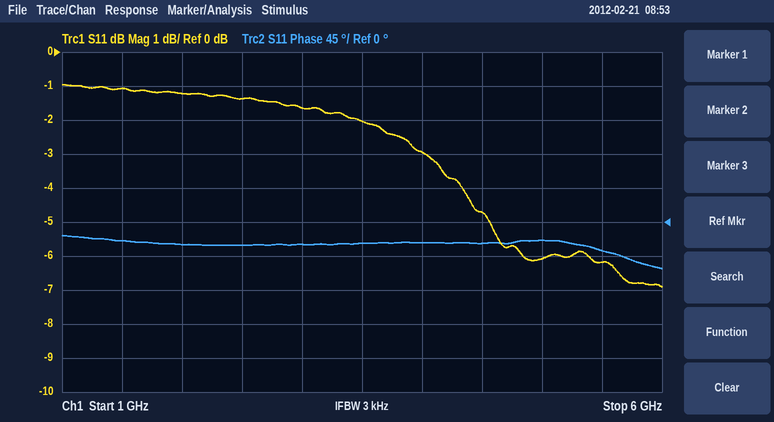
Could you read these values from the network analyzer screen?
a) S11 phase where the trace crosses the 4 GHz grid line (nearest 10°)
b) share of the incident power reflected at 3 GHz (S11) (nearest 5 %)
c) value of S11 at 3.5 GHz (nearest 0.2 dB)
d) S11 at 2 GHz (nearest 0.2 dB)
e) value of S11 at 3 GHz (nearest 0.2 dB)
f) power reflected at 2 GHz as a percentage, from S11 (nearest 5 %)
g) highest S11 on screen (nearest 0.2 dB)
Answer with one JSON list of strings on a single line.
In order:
["-30°", "70 %", "-2.0 dB", "-1.2 dB", "-1.6 dB", "75 %", "-1.0 dB"]
